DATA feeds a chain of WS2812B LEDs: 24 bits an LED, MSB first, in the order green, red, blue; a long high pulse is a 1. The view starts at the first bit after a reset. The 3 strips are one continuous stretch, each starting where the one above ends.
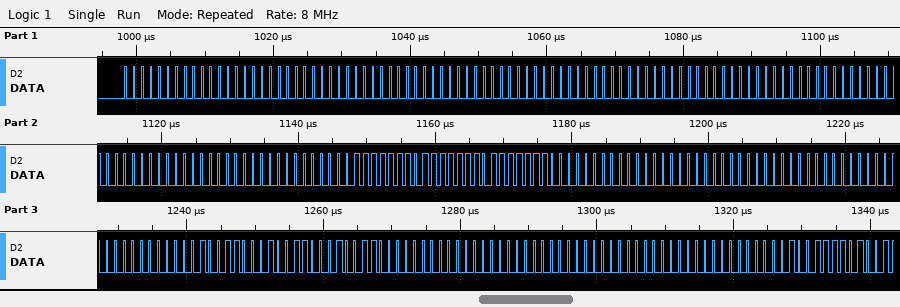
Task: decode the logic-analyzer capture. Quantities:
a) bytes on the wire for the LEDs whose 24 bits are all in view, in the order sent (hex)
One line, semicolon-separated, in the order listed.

00 00 00 00 00 00 00 00 00 00 00 00 00 00 00 FE FE FE 00 00 00 00 00 00 13 13 13 00 00 00 00 00 00
